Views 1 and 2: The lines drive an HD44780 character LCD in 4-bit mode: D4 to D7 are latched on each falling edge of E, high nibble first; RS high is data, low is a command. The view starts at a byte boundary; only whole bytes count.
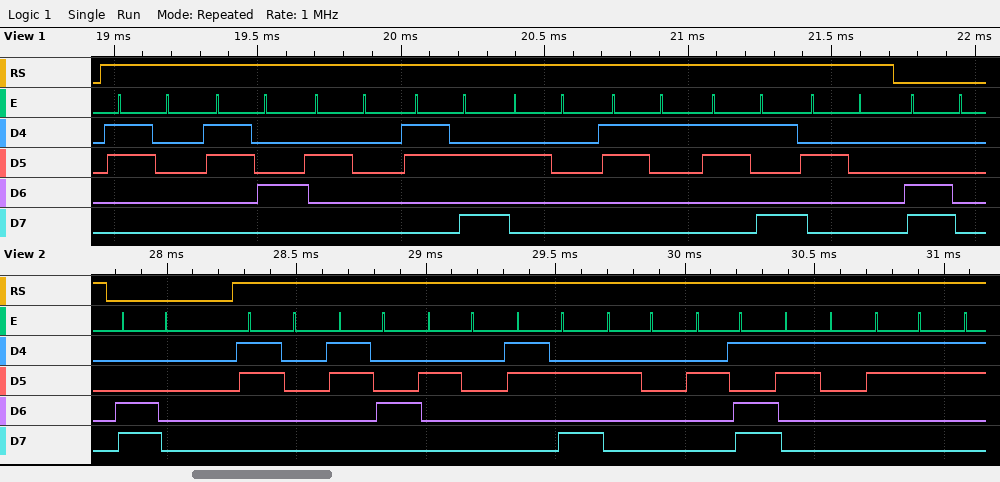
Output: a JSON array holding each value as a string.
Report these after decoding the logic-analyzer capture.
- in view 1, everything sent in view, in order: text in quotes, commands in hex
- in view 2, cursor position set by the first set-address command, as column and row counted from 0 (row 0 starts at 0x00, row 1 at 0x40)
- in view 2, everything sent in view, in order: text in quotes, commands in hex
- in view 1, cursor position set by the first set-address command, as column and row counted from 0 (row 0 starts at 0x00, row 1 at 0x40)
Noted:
["\"04 : 19 \" 0xC0", "column 0, row 1", "0xC0 \"04 : -13\"", "column 0, row 1"]
